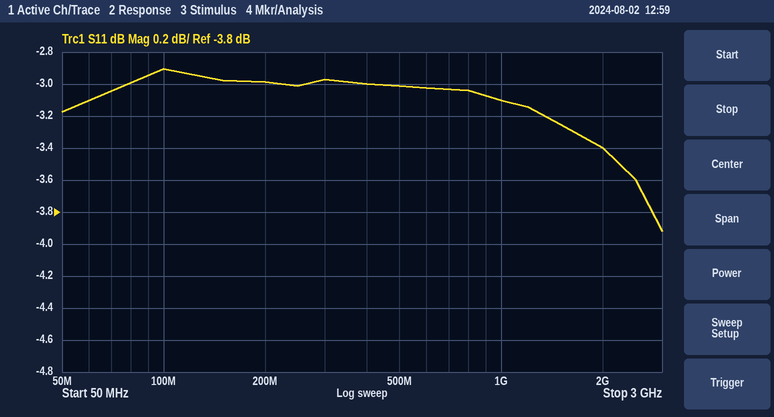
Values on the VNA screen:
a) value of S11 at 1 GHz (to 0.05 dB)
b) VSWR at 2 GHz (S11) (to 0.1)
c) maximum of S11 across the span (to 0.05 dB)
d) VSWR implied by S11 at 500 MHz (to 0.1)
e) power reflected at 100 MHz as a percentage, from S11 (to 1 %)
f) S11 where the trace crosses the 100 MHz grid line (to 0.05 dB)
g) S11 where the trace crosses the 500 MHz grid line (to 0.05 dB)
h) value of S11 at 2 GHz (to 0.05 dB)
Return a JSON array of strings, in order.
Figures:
["-3.10 dB", "5.2", "-2.90 dB", "5.8", "51 %", "-2.90 dB", "-3.00 dB", "-3.40 dB"]
